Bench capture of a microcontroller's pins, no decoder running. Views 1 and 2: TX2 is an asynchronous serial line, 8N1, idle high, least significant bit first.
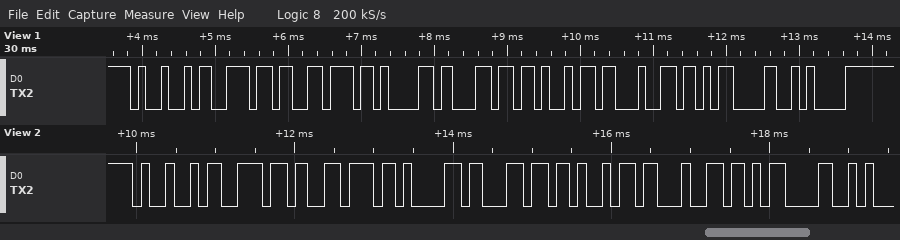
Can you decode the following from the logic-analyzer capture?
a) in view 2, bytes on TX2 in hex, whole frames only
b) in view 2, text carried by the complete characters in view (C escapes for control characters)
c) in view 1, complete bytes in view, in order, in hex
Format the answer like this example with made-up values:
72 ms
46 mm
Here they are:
49 6E 76 61 6C 69 64 0D
"Invalid\r"
0x49 0x6E 0x76 0x61 0x6C 0x69 0x64 0x0D 0x0A
